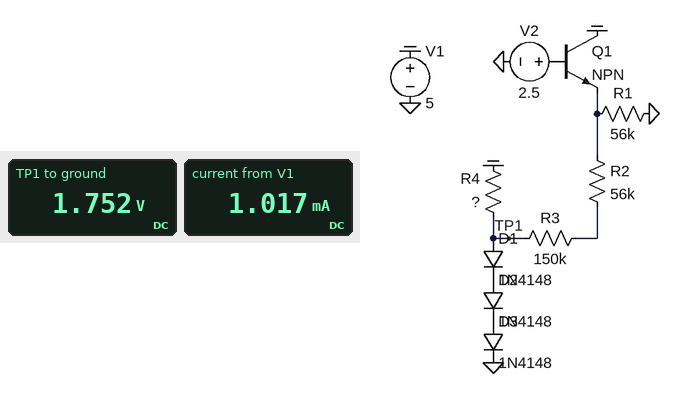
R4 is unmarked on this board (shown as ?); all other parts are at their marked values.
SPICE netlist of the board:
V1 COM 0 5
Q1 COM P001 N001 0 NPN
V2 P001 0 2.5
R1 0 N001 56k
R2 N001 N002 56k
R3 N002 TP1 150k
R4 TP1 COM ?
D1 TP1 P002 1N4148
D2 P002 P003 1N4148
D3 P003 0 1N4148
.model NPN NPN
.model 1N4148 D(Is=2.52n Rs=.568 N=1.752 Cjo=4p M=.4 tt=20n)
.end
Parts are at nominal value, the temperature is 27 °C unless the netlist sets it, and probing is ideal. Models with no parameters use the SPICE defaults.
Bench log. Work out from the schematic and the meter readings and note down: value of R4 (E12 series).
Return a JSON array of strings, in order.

["3.3 kΩ"]
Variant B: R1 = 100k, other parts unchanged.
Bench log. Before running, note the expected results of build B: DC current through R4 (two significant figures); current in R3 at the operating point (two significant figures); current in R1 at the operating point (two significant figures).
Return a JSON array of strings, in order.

["980 µA", "370 nA", "18 µA"]
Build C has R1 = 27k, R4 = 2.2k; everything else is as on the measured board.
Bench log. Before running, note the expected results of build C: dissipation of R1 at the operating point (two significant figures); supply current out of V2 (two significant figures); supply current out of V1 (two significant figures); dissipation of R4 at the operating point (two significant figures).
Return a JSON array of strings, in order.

["120 µW", "660 nA", "1.5 mA", "4.6 mW"]
